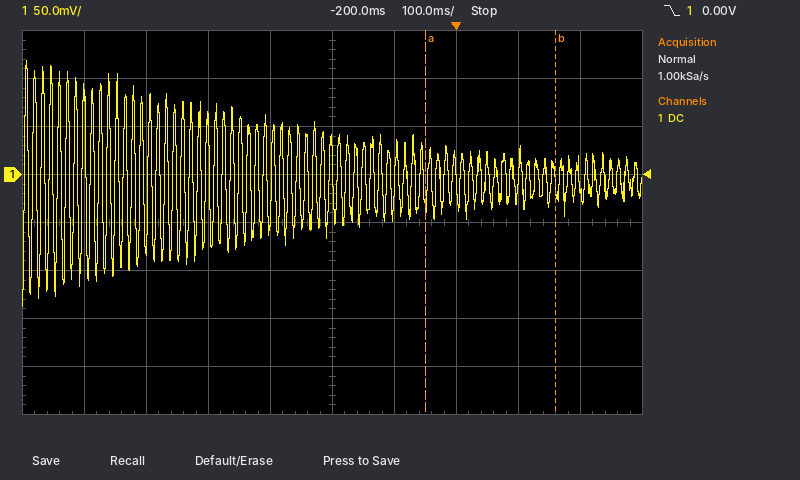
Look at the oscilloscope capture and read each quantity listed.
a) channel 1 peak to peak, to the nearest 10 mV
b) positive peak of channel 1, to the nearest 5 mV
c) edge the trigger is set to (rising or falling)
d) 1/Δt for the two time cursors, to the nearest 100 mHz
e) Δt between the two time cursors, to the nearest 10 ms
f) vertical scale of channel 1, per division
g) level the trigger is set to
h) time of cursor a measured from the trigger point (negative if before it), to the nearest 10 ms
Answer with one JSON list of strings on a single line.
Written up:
["260 mV", "120 mV", "falling", "4.8 Hz", "210 ms", "50 mV", "0.00 V", "-50 ms"]
